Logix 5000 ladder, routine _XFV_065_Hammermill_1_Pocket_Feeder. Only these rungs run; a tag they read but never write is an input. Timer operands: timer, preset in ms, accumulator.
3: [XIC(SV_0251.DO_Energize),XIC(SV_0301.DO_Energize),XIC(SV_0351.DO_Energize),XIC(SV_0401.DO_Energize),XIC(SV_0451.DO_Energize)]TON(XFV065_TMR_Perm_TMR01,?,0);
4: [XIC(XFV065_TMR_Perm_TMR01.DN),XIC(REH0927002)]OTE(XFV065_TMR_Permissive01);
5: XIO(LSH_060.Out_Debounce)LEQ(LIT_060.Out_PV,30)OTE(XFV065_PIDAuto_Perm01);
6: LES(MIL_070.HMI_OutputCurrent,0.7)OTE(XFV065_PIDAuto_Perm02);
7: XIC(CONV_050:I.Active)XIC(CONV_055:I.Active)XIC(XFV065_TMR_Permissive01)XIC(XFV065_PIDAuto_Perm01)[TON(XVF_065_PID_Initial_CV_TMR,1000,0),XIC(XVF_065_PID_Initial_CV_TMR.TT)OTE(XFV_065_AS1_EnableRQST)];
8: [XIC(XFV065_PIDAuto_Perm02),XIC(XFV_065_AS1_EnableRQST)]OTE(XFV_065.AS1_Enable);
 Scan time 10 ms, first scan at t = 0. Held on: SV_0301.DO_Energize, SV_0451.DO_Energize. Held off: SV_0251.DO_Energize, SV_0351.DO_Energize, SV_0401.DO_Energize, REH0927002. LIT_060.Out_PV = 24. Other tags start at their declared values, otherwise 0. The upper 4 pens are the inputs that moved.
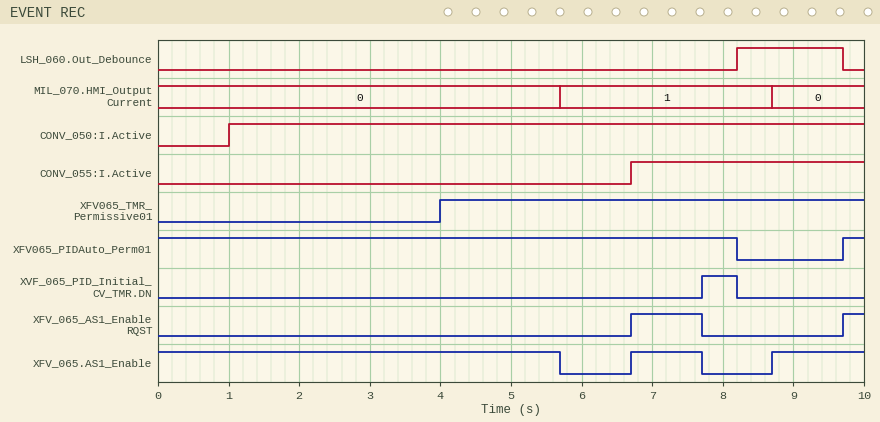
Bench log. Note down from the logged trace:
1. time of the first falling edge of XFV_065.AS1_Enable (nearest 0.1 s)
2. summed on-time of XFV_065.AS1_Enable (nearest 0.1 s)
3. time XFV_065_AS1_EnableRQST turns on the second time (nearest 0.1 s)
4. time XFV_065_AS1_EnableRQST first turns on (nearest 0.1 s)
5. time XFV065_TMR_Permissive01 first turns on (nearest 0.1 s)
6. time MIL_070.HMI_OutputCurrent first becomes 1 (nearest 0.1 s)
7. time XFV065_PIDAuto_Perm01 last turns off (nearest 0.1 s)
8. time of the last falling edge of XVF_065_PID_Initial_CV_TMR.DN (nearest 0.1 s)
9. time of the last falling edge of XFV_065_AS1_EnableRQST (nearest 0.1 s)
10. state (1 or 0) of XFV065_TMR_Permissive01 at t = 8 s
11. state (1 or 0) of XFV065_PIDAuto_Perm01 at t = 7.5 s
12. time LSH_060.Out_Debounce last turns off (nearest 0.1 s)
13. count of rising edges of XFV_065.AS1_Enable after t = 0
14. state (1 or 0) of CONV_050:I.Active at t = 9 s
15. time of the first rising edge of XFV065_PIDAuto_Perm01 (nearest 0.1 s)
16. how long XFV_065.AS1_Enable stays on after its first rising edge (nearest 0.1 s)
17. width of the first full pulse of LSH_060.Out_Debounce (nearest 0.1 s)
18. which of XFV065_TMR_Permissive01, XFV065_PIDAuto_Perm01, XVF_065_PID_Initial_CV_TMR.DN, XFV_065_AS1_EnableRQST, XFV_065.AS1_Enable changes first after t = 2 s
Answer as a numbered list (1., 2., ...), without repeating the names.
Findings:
1. 5.7 s
2. 8.0 s
3. 9.7 s
4. 6.7 s
5. 4.0 s
6. 5.7 s
7. 8.2 s
8. 8.2 s
9. 7.7 s
10. 1
11. 1
12. 9.7 s
13. 2
14. 1
15. 9.7 s
16. 1.0 s
17. 1.5 s
18. XFV065_TMR_Permissive01
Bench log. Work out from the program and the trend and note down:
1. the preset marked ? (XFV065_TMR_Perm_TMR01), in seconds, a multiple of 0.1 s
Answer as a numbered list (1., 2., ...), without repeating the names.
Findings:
1. 4.0 s
